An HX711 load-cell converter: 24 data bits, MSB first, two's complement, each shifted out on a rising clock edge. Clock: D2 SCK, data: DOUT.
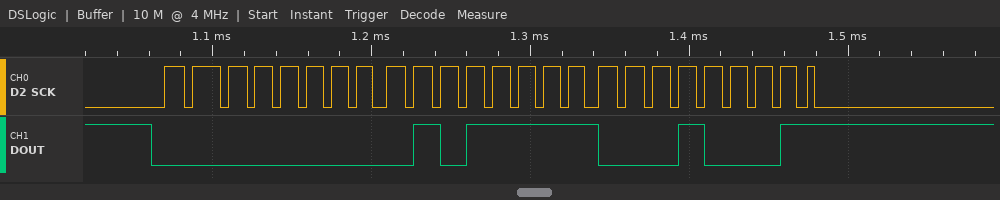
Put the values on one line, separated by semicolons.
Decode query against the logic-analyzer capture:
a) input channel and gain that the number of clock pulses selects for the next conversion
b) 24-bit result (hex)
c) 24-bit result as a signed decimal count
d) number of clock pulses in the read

channel A, gain 128; 0x005F11; 24337; 25
